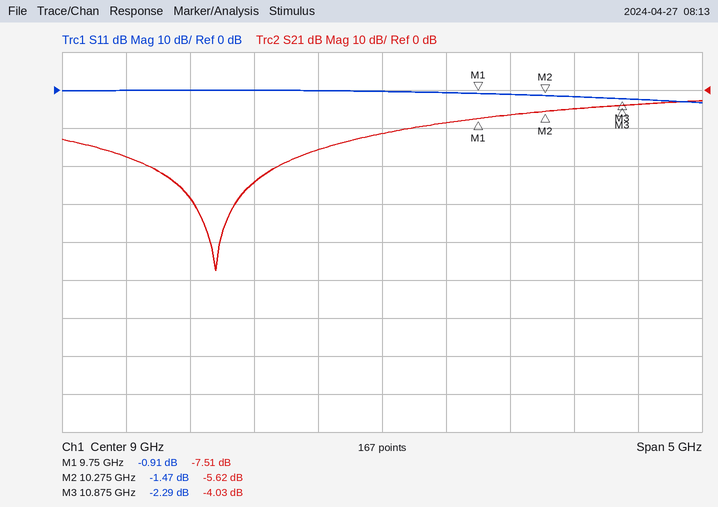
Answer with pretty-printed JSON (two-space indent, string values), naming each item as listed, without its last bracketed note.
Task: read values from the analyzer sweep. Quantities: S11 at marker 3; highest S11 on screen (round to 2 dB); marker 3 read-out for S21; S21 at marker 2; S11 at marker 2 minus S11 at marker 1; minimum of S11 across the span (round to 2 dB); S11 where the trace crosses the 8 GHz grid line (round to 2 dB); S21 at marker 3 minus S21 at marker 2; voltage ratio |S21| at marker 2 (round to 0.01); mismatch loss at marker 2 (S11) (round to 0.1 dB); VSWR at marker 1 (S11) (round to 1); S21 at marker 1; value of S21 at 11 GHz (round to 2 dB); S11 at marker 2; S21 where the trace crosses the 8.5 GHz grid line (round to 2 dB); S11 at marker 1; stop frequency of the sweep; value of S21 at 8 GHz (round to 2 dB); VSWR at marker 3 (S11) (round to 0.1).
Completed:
{
  "S11 at marker 3": "-2.29 dB",
  "highest S11 on screen": "0 dB",
  "marker 3 read-out for S21": "-4.03 dB",
  "S21 at marker 2": "-5.62 dB",
  "S11 at marker 2 minus S11 at marker 1": "-0.56 dB",
  "minimum of S11 across the span": "-4 dB",
  "S11 where the trace crosses the 8 GHz grid line": "0 dB",
  "S21 at marker 3 minus S21 at marker 2": "1.59 dB",
  "voltage ratio |S21| at marker 2": "0.52",
  "mismatch loss at marker 2 (S11)": "5.4 dB",
  "VSWR at marker 1 (S11)": "19",
  "S21 at marker 1": "-7.51 dB",
  "value of S21 at 11 GHz": "-4 dB",
  "S11 at marker 2": "-1.47 dB",
  "S21 where the trace crosses the 8.5 GHz grid line": "-16 dB",
  "S11 at marker 1": "-0.91 dB",
  "stop frequency of the sweep": "11.5 GHz",
  "value of S21 at 8 GHz": "-24 dB",
  "VSWR at marker 3 (S11)": "7.6"
}
